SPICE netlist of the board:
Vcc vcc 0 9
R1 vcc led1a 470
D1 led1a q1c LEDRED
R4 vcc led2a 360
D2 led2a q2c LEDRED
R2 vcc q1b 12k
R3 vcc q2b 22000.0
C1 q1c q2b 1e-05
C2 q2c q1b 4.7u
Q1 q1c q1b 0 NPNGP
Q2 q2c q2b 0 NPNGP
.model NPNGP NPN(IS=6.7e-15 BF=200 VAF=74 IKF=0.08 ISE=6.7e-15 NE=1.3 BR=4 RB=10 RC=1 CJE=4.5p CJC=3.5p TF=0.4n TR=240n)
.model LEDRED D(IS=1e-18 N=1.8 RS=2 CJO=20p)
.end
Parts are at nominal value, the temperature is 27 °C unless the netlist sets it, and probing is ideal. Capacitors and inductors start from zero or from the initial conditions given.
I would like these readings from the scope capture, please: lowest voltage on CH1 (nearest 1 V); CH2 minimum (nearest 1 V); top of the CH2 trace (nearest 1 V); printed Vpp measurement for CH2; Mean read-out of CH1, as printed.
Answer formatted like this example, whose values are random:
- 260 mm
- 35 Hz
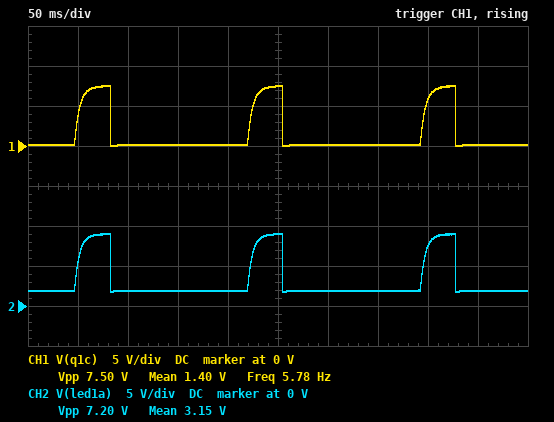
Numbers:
- 0 V
- 2 V
- 9 V
- 7.20 V
- 1.40 V
